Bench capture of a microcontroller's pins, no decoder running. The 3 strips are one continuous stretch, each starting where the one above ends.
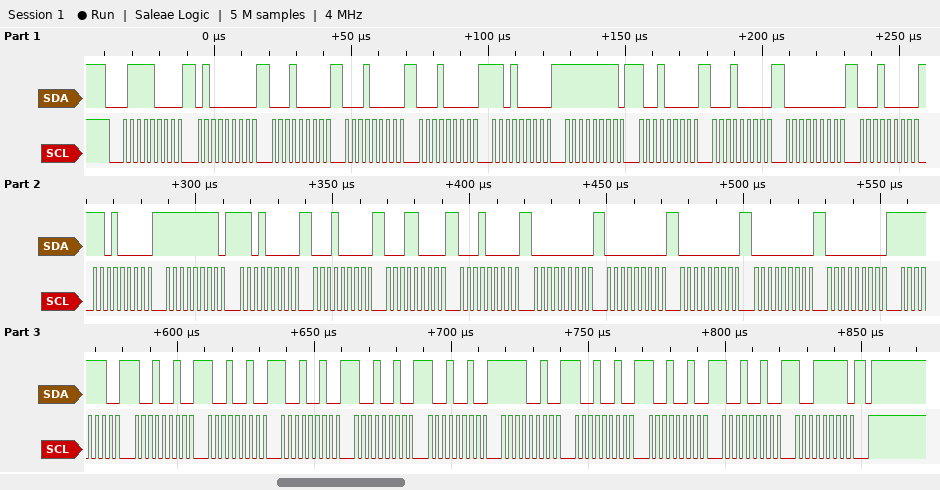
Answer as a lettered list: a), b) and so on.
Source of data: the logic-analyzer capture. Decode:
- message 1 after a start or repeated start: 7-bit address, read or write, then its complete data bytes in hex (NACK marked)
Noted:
a) 0x3C write: 40 10 10 10 D0 FF 90 10 00 10 D0 FF D0 10 18 10 00 00 00 00 00 FE 92 92 92 92 92 F2 92 92 92 9F
